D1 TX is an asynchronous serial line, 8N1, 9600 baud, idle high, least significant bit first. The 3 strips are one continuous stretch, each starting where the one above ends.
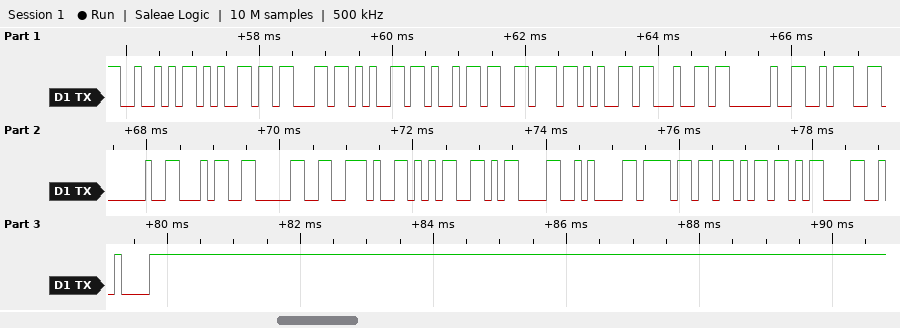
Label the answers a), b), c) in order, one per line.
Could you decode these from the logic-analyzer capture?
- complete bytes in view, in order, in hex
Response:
a) 52 65 63 65 69 76 65 64 20 3A 20 34 30 2E 35 0D 0A 6F 6B 0D 0A
